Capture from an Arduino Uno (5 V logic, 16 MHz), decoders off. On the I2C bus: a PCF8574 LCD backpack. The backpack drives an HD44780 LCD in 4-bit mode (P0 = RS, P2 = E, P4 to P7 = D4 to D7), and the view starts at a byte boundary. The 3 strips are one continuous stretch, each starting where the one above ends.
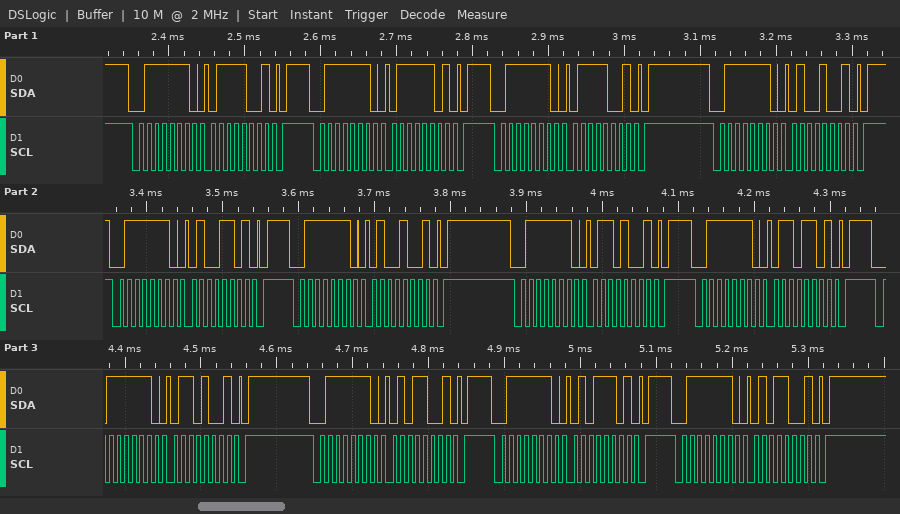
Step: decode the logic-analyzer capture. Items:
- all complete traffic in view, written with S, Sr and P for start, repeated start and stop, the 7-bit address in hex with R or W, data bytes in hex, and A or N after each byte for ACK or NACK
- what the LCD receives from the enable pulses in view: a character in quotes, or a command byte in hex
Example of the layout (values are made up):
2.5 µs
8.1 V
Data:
S 3FW A 79 A P S 3FW A 7D A P S 3FW A 79 A P S 3FW A 49 A P S 3FW A 4D A P S 3FW A 49 A P S 3FW A 69 A P S 3FW A 6D A P S 3FW A 69 A P S 3FW A 59 A P S 3FW A 5D A P S 3FW A 59 A P
't' 'e'
